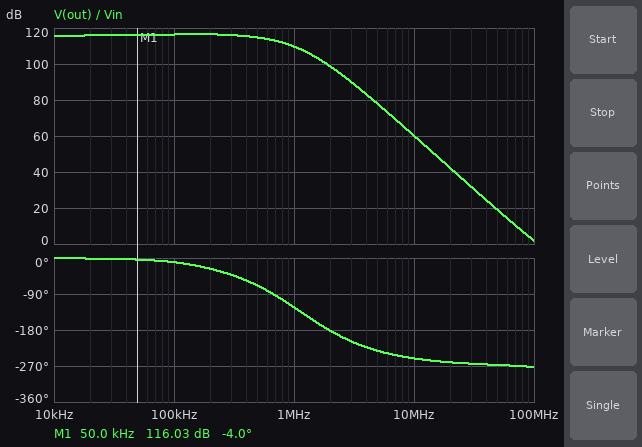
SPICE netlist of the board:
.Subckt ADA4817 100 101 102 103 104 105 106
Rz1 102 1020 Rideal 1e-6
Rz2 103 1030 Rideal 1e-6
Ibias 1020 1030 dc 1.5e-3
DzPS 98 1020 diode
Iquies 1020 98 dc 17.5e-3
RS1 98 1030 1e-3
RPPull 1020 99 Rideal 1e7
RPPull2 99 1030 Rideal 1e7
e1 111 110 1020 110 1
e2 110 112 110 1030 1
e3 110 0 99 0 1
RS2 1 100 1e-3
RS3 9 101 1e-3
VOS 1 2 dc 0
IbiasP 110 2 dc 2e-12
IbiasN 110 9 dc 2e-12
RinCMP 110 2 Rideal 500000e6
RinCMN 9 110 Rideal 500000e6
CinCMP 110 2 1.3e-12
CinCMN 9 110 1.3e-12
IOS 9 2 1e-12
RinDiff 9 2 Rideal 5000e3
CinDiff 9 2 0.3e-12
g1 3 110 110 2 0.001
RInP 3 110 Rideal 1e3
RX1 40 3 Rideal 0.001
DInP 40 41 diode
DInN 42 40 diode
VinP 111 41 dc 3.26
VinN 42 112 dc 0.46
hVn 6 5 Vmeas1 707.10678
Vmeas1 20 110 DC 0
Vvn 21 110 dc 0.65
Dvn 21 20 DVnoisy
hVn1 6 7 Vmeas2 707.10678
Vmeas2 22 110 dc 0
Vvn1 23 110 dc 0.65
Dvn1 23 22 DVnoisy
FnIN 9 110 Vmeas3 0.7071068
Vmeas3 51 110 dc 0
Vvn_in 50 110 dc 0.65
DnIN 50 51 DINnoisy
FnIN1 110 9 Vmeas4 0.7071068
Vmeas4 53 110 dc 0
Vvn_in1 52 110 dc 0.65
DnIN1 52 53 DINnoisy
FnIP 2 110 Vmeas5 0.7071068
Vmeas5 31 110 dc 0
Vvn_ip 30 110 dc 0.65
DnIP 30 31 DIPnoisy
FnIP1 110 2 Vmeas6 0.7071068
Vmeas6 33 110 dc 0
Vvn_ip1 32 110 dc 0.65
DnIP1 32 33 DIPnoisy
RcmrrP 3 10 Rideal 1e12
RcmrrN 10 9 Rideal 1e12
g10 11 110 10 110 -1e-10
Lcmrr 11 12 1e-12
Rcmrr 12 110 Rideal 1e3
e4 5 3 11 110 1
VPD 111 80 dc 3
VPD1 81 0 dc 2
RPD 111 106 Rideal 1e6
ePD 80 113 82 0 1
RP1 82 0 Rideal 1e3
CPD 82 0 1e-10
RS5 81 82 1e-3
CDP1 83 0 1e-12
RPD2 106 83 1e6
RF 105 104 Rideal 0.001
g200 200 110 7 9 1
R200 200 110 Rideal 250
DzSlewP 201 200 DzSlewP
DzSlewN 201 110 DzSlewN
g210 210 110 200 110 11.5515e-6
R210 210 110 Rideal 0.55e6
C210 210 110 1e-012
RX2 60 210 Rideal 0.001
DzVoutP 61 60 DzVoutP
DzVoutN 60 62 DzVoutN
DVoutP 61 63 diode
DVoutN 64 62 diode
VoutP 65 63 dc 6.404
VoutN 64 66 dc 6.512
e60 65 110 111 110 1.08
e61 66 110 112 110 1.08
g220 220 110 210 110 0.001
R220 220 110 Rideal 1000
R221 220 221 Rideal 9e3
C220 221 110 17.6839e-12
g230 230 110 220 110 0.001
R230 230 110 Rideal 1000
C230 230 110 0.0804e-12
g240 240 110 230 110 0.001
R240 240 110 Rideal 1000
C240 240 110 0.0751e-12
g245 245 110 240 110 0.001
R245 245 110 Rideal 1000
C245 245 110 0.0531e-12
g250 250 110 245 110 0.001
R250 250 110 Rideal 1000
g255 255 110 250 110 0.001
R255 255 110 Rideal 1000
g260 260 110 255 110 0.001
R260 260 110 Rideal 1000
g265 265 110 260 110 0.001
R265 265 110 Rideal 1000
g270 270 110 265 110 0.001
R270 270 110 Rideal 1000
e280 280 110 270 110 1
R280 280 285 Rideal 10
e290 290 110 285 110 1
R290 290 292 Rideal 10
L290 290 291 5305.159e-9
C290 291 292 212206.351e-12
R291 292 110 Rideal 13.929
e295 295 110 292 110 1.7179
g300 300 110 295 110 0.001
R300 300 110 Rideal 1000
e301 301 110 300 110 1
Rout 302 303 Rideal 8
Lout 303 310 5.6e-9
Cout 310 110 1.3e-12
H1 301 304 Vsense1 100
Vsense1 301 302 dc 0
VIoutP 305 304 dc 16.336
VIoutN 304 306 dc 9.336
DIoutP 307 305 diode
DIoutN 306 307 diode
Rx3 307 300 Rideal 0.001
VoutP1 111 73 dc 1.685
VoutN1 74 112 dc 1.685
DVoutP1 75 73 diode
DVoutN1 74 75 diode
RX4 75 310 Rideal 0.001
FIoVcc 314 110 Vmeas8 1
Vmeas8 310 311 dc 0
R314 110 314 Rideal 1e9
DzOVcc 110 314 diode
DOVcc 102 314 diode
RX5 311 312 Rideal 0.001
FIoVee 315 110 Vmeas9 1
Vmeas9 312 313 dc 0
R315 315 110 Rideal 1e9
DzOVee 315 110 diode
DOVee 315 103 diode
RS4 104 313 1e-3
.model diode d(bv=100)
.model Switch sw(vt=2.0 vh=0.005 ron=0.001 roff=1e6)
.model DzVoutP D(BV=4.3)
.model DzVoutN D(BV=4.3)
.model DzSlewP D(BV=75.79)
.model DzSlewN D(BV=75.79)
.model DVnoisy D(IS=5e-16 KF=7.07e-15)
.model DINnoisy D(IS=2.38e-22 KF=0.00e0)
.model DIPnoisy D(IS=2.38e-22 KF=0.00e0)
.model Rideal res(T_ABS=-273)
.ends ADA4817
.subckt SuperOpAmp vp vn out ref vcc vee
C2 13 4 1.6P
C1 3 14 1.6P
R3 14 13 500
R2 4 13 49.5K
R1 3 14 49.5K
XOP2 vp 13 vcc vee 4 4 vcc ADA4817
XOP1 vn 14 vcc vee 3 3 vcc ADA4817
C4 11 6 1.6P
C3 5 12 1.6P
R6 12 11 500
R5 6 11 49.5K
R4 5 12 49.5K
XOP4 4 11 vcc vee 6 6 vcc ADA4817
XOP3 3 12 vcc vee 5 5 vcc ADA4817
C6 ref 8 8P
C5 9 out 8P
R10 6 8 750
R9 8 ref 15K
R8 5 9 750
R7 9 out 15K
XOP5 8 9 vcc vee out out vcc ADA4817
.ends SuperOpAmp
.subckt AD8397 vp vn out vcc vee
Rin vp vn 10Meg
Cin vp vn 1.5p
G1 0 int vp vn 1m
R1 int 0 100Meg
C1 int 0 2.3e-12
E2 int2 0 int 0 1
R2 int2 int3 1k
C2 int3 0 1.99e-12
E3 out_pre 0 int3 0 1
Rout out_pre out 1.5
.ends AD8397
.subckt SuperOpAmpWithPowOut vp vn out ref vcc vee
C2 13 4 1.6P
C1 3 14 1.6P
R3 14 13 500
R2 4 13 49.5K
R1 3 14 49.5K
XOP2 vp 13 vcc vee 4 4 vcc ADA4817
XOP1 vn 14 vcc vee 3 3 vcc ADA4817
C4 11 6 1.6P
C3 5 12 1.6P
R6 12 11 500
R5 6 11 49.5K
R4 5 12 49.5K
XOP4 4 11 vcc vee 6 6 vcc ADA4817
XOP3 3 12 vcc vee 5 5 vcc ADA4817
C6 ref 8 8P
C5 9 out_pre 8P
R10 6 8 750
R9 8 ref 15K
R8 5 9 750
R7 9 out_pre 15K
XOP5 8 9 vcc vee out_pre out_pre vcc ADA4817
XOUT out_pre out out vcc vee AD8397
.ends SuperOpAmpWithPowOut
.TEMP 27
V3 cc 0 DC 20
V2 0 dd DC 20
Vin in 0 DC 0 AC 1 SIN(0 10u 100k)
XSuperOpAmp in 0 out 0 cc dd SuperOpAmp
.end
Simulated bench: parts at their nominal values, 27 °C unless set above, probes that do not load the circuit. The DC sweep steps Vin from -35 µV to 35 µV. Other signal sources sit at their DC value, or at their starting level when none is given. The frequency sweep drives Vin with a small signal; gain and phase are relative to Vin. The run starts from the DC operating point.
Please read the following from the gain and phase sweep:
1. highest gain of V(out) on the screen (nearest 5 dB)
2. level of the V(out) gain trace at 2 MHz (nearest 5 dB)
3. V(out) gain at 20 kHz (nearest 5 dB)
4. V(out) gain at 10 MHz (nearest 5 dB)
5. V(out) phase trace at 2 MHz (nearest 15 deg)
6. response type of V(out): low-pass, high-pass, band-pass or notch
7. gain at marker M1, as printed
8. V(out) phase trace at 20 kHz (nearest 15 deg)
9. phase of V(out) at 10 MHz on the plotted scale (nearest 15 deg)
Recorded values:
115 dB
100 dB
115 dB
60 dB
-180 deg
low-pass
116.03 dB
0 deg
-255 deg
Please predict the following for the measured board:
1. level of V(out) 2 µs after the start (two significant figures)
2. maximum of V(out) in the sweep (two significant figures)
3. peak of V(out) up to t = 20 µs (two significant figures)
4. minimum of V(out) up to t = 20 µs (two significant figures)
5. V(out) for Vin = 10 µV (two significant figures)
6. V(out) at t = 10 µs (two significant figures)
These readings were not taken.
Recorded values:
5.6 V
19 V
6.6 V
-6.6 V
6.2 V
-1.2 V
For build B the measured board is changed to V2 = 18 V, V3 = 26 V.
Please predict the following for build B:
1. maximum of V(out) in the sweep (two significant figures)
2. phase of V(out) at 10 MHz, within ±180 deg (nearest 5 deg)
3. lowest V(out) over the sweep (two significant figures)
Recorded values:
22 V
110 deg
-17 V
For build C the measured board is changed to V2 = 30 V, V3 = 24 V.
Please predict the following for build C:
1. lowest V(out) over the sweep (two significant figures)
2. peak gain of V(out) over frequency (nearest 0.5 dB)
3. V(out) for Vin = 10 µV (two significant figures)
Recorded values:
-22 V
116.5 dB
6.1 V
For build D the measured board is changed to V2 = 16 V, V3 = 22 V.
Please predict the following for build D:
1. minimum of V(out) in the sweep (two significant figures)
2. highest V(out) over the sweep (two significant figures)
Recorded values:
-15 V
21 V
